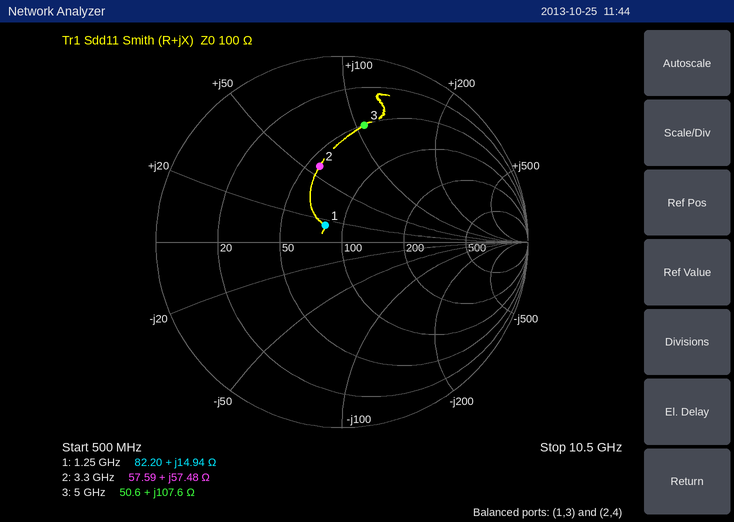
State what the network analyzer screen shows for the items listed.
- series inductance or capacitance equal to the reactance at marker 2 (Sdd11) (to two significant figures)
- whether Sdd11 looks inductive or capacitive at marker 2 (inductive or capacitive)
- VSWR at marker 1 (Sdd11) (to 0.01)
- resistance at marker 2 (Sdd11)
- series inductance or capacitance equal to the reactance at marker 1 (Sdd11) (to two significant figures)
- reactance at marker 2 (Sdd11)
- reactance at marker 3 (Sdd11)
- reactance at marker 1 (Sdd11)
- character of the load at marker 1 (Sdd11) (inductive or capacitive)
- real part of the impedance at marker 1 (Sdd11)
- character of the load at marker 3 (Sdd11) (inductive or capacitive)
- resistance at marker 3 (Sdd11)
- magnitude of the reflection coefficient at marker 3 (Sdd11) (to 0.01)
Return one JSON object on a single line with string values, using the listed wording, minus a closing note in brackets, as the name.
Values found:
{"series inductance or capacitance equal to the reactance at marker 2 (Sdd11)": "2.8 nH", "whether Sdd11 looks inductive or capacitive at marker 2": "inductive", "VSWR at marker 1 (Sdd11)": "1.29", "resistance at marker 2": "57.59 Ω", "series inductance or capacitance equal to the reactance at marker 1 (Sdd11)": "1.9 nH", "reactance at marker 2": "+57.48 Ω", "reactance at marker 3": "+107.6 Ω", "reactance at marker 1": "+14.94 Ω", "character of the load at marker 1 (Sdd11)": "inductive", "real part of the impedance at marker 1": "82.20 Ω", "character of the load at marker 3 (Sdd11)": "inductive", "resistance at marker 3": "50.6 Ω", "magnitude of the reflection coefficient at marker 3 (Sdd11)": "0.64"}
